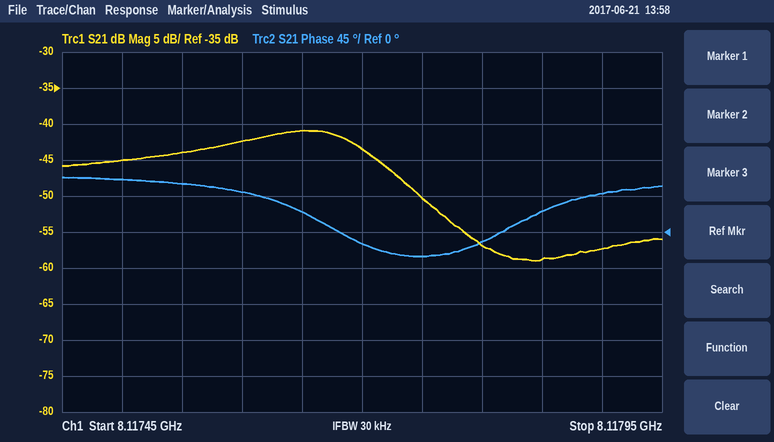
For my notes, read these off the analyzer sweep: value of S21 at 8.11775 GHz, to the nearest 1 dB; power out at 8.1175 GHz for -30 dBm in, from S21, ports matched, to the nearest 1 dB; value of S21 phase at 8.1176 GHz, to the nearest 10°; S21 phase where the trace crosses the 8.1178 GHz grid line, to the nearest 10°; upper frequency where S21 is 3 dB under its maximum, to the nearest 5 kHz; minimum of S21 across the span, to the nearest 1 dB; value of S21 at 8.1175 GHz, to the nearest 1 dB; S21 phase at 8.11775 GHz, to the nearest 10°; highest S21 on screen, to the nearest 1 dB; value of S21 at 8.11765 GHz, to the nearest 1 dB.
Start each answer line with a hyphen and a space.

- -50 dB
- -75 dBm
- 50°
- -10°
- 8.117705 GHz
- -59 dB
- -45 dB
- -30°
- -41 dB
- -41 dB
